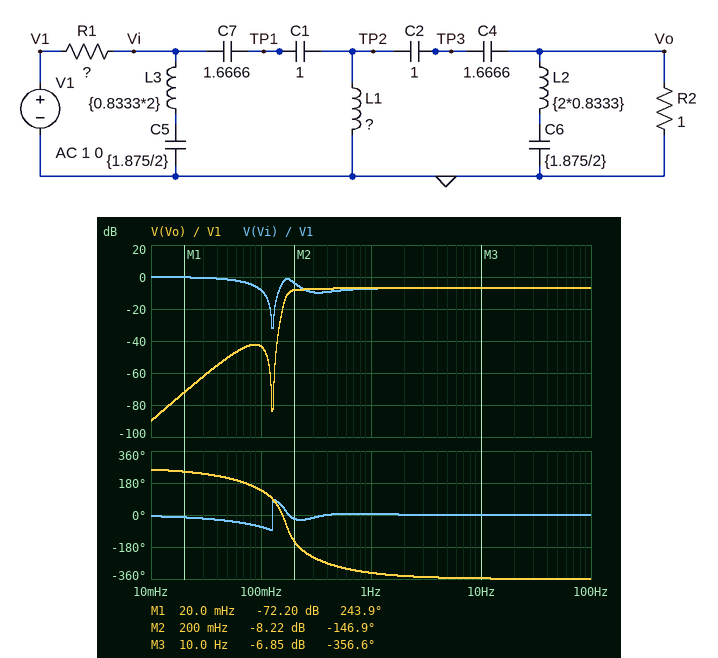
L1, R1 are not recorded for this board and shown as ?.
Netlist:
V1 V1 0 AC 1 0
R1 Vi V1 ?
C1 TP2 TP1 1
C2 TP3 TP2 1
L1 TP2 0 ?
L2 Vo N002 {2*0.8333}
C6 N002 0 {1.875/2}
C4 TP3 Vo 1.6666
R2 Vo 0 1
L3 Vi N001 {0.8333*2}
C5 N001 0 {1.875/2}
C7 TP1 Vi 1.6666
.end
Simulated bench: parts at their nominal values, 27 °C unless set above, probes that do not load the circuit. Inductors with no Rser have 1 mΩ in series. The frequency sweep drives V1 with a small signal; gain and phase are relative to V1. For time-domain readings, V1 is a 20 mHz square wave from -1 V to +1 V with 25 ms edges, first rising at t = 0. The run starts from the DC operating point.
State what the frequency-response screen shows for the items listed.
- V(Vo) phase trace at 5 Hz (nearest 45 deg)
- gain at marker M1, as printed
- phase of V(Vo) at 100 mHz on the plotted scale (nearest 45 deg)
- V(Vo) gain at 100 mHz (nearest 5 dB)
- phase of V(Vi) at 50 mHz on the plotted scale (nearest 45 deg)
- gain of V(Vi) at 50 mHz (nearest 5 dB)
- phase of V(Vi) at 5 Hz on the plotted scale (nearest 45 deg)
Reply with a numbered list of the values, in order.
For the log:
1. -360 deg
2. -72.20 dB
3. 135 deg
4. -45 dB
5. -45 deg
6. 0 dB
7. 0 deg
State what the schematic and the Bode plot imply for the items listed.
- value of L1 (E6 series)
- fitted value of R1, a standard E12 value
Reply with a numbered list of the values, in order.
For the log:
1. 330 mH
2. 1.2 Ω
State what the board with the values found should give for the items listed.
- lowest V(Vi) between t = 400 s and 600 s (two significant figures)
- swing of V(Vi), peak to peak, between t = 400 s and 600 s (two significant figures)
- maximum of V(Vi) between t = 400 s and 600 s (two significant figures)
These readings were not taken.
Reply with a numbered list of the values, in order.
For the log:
1. -1.2 V
2. 2.4 V
3. 1.2 V
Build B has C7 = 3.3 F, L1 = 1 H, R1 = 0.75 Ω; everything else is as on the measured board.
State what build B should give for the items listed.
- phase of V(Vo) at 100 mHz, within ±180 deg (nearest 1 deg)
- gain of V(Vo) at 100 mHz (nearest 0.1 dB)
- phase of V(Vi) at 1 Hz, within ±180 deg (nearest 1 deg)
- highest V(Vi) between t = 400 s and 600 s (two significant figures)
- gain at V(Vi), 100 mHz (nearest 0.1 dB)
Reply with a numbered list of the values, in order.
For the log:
1. 145 deg
2. -25.1 dB
3. -2 deg
4. 1.2 V
5. -6.1 dB
